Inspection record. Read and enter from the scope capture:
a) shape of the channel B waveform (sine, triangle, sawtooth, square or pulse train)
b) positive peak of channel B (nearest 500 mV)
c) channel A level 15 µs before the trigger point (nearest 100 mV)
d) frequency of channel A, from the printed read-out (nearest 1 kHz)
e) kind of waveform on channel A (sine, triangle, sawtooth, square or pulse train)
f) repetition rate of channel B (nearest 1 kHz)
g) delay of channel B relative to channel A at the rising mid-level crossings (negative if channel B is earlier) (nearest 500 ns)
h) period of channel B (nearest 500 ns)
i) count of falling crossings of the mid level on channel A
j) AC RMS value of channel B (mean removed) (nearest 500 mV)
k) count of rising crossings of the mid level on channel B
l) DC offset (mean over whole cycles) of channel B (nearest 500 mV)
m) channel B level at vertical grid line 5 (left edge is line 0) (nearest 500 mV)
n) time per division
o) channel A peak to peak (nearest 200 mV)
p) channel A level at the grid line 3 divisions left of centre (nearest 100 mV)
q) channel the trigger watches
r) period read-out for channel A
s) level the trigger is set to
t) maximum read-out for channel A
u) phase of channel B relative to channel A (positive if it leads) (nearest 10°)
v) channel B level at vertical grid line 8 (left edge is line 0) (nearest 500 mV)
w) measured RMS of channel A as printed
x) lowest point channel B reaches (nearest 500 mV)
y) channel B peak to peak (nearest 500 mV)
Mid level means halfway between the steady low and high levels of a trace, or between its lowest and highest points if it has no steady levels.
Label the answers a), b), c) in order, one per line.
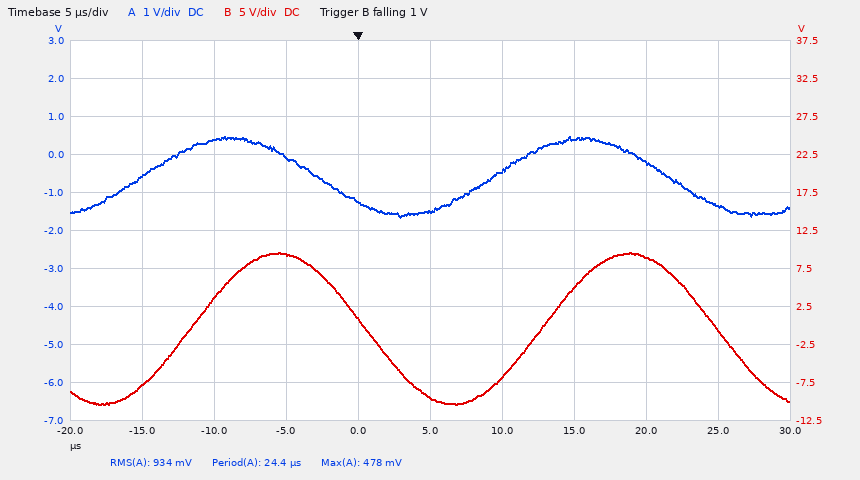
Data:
a) sine
b) 9.5 V
c) -600 mV
d) 41 kHz
e) sine
f) 41 kHz
g) +3.5 µs
h) 24.5 µs
i) 2
j) 7.0 V
k) 2
l) -500 mV
m) -9.5 V
n) 5 µs
o) 2.2 V
p) 400 mV
q) channel B
r) 24.4 µs
s) 1 V
t) 478 mV
u) -50°
v) 9.0 V
w) 934 mV
x) -10.5 V
y) 20.0 V
